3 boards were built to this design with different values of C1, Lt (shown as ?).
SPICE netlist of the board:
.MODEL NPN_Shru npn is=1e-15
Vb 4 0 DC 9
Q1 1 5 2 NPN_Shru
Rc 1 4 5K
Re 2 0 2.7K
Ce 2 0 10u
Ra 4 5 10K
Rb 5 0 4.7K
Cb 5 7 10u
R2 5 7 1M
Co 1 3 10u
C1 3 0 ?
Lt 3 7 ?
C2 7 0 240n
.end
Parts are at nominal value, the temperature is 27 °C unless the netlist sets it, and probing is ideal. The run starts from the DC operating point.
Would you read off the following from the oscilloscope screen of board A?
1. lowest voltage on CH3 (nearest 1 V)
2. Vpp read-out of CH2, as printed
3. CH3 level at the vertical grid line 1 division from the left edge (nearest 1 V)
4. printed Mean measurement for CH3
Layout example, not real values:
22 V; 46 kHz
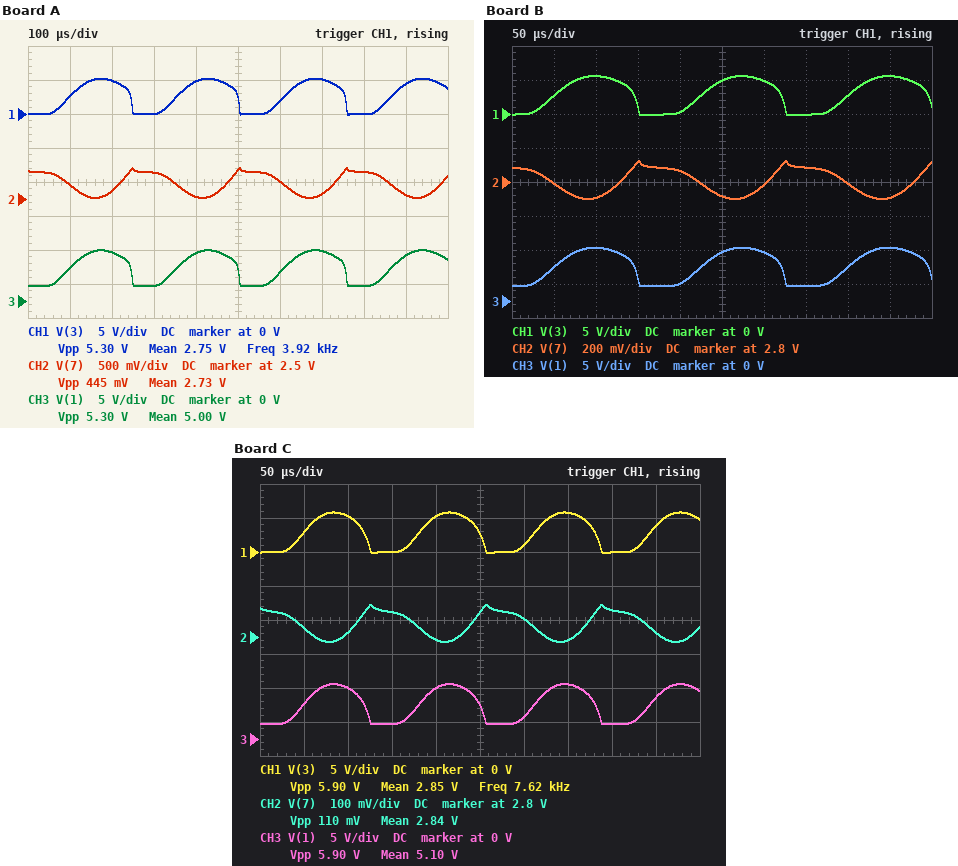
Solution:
2 V; 445 mV; 5 V; 5.00 V
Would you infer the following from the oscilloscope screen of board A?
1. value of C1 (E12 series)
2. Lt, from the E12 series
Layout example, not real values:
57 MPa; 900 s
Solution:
33 nF; 82 mH
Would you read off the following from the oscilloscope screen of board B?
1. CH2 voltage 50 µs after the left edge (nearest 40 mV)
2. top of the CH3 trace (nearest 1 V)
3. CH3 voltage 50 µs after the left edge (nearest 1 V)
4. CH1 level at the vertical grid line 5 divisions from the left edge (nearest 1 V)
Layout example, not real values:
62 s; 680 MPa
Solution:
2.80 V; 8 V; 5 V; 5 V
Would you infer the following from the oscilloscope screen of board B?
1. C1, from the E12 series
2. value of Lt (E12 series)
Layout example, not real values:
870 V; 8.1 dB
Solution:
15 nF; 82 mH
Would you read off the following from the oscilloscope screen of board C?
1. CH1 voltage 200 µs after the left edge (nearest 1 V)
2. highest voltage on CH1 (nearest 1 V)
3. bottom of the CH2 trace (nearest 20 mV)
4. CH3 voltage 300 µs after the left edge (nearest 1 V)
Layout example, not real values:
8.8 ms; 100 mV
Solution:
5 V; 6 V; 2.78 V; 3 V
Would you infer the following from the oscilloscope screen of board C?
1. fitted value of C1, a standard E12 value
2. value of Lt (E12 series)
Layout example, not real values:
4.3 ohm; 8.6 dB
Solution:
6.8 nF; 100 mH
